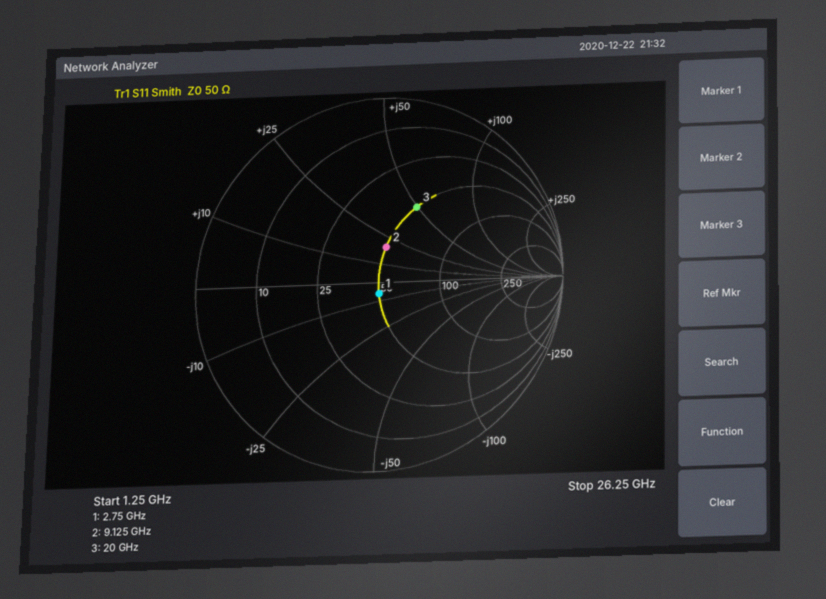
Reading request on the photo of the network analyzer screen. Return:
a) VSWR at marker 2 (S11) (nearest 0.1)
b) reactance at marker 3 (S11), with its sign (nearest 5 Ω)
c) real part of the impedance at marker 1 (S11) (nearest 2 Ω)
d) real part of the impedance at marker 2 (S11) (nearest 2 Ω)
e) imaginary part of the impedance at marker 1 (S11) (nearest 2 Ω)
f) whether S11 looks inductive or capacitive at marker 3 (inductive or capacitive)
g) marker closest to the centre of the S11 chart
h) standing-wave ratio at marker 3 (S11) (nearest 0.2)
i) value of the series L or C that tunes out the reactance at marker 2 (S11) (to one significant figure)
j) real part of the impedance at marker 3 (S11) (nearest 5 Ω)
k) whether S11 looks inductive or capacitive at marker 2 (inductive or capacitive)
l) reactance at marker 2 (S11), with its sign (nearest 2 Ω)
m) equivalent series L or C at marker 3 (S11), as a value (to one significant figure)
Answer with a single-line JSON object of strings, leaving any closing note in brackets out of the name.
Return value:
{"VSWR at marker 2 (S11)": "1.5", "reactance at marker 3 (S11), with its sign": "+50 Ω", "real part of the impedance at marker 1 (S11)": "50 Ω", "real part of the impedance at marker 2 (S11)": "50 Ω", "imaginary part of the impedance at marker 1 (S11)": "-6 Ω", "whether S11 looks inductive or capacitive at marker 3": "inductive", "marker closest to the centre of the S11 chart": "marker 1", "standing-wave ratio at marker 3 (S11)": "2.6", "value of the series L or C that tunes out the reactance at marker 2 (S11)": "900 fF", "real part of the impedance at marker 3 (S11)": "50 Ω", "whether S11 looks inductive or capacitive at marker 2": "inductive", "reactance at marker 2 (S11), with its sign": "+20 Ω", "equivalent series L or C at marker 3 (S11), as a value": "400 pH"}
